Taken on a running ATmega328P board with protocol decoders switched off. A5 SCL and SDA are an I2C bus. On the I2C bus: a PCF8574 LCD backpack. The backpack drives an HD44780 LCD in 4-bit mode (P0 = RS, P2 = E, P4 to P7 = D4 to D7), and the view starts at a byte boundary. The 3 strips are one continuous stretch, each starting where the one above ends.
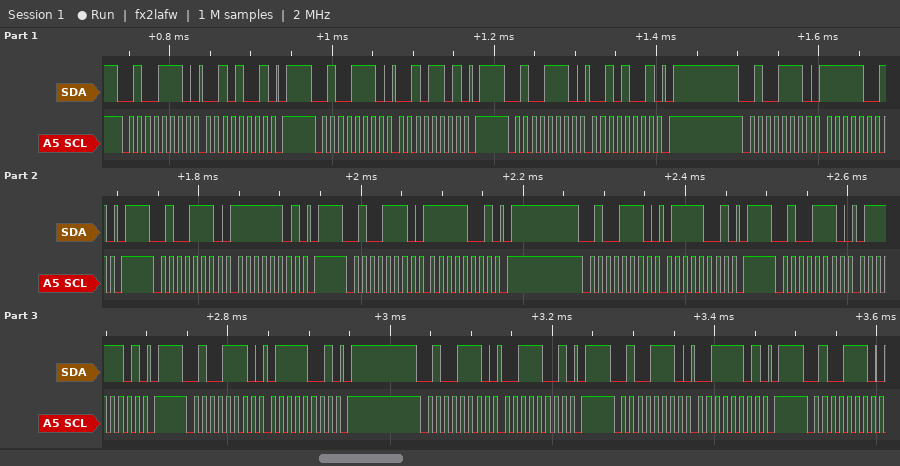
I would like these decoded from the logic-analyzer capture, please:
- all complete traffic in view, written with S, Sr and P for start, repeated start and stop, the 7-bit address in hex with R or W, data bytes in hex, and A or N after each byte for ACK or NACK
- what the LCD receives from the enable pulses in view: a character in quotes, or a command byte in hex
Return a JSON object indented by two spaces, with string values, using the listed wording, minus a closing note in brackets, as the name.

{
  "all complete traffic in view, written with S, Sr and P for start, repeated start and stop, the 7-bit address in hex with R or W, data bytes in hex, and A or N after each byte for ACK or NACK": "S 27W A 29 A P S 27W A 2D A P S 27W A 29 A P S 27W A F9 A P S 27W A FD A P S 27W A F9 A P S 27W A 79 A P S 27W A 7D A P S 27W A 79 A P S 27W A 39 A P S 27W A 3D A P S 27W A",
  "what the LCD receives from the enable pulses in view: a character in quotes, or a command byte in hex": "'/'"
}
